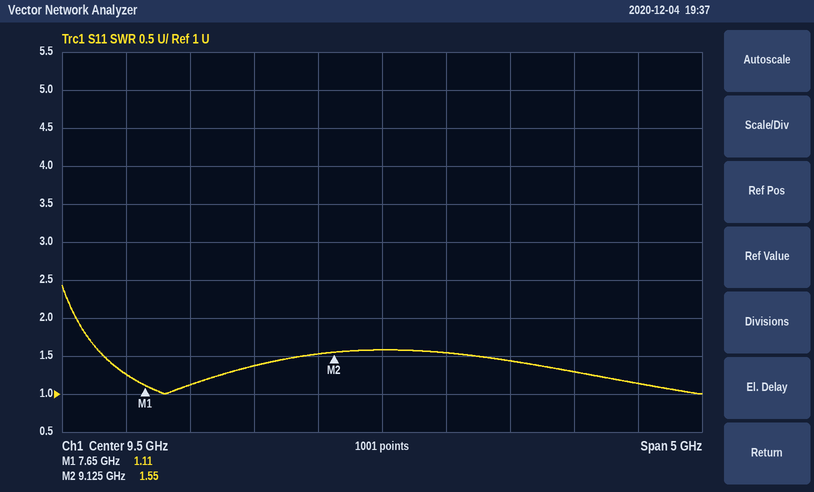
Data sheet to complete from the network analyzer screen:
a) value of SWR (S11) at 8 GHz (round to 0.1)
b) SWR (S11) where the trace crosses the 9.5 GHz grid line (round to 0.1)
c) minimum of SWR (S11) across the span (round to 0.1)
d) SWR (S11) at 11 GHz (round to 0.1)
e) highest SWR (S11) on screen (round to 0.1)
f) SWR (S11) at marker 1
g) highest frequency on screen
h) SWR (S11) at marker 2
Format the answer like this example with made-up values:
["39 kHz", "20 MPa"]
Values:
["1.1", "1.6", "1.0", "1.3", "2.4", "1.11", "12 GHz", "1.55"]
